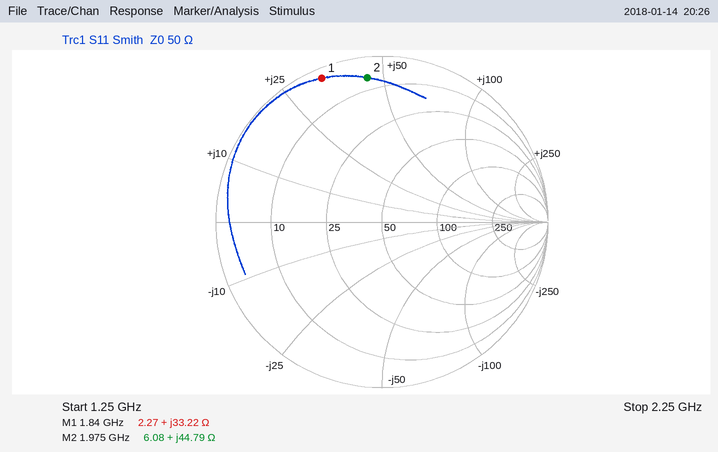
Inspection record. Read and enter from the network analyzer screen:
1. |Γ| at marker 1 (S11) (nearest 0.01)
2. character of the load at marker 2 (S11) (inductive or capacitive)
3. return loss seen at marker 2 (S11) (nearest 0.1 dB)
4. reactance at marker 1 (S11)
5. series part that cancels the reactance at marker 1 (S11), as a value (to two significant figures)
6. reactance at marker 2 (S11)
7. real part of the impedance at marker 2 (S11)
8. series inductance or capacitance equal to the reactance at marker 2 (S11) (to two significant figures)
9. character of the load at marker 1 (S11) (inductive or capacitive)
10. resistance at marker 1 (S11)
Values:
0.94
inductive
1.2 dB
+33.22 Ω
2.6 pF
+44.79 Ω
6.08 Ω
3.6 nH
inductive
2.27 Ω
